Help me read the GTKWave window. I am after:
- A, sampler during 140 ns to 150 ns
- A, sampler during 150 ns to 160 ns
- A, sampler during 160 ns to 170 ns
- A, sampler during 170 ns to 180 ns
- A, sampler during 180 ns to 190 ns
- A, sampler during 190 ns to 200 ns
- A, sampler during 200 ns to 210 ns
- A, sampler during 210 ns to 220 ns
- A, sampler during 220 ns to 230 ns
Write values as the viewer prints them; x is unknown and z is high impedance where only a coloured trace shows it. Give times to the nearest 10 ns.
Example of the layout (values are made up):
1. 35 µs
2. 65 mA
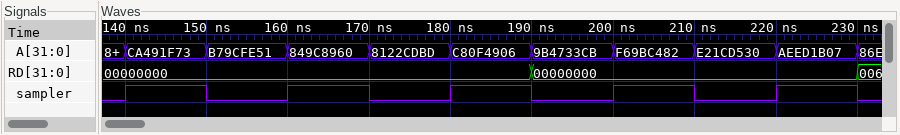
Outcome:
1. A=CA491F73, sampler=1
2. A=B79CFE51, sampler=0
3. A=849C8960, sampler=1
4. A=8122CDBD, sampler=0
5. A=C80F4906, sampler=1
6. A=9B4733CB, sampler=0
7. A=F69BC482, sampler=1
8. A=E21CD530, sampler=0
9. A=AEED1B07, sampler=1
